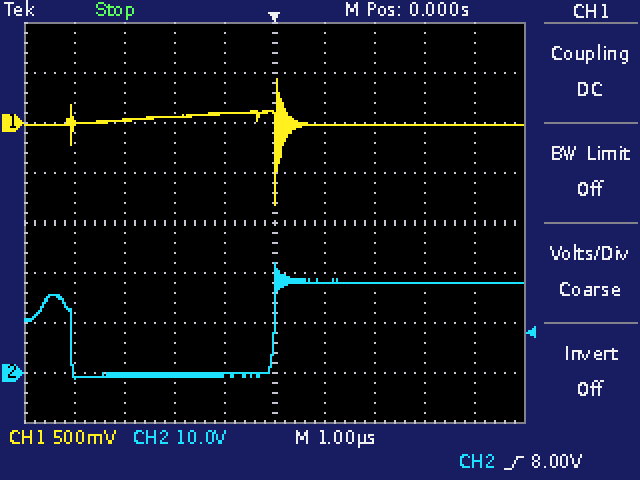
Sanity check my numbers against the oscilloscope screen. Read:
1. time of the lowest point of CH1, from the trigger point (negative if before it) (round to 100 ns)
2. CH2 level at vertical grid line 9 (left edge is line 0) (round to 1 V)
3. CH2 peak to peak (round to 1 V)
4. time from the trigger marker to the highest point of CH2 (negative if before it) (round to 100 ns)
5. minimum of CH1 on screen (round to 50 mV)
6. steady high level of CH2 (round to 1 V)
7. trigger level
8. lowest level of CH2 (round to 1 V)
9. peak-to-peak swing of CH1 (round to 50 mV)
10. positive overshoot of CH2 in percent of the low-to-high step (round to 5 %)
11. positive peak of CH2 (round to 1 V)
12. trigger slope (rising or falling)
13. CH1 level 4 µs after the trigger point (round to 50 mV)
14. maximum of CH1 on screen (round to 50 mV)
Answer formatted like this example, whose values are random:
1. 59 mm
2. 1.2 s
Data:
1. 0.0 µs
2. 18 V
3. 23 V
4. 0.0 µs
5. -800 mV
6. 18 V
7. 8.00 V
8. -1 V
9. 1.25 V
10. 20 %
11. 22 V
12. rising
13. 0 mV
14. 450 mV
